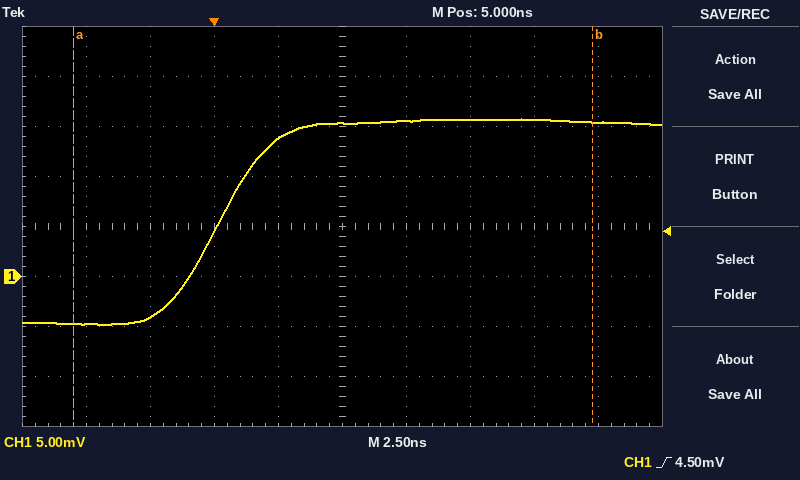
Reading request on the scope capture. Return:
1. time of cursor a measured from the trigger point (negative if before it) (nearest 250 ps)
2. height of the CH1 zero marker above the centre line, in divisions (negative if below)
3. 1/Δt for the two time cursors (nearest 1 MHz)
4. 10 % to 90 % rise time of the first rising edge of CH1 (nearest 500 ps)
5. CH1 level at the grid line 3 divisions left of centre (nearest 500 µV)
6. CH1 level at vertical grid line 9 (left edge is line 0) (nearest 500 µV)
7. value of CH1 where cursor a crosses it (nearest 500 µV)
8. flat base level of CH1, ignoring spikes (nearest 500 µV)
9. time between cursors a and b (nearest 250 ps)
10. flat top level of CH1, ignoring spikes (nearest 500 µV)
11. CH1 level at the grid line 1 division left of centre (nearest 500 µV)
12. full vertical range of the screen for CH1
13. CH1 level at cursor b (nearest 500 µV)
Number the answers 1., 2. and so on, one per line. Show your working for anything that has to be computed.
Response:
1. -5.50 ns
2. -1.0 div
3. 1 / 20.25 ns ≈ 49 MHz
4. 4.0 ns
5. -4.0 mV
6. 15.5 mV
7. -4.5 mV
8. -4.5 mV
9. 20.25 ns
10. 15.5 mV
11. 14.0 mV
12. 40 mV
13. 15.5 mV
